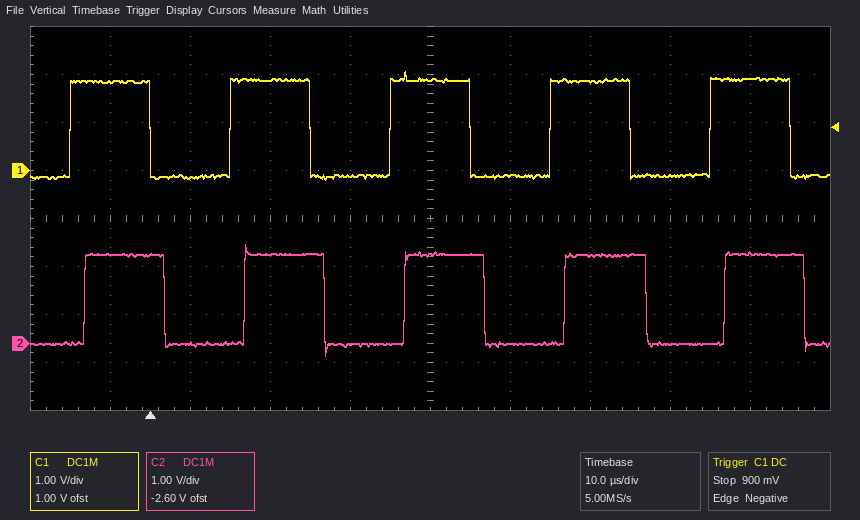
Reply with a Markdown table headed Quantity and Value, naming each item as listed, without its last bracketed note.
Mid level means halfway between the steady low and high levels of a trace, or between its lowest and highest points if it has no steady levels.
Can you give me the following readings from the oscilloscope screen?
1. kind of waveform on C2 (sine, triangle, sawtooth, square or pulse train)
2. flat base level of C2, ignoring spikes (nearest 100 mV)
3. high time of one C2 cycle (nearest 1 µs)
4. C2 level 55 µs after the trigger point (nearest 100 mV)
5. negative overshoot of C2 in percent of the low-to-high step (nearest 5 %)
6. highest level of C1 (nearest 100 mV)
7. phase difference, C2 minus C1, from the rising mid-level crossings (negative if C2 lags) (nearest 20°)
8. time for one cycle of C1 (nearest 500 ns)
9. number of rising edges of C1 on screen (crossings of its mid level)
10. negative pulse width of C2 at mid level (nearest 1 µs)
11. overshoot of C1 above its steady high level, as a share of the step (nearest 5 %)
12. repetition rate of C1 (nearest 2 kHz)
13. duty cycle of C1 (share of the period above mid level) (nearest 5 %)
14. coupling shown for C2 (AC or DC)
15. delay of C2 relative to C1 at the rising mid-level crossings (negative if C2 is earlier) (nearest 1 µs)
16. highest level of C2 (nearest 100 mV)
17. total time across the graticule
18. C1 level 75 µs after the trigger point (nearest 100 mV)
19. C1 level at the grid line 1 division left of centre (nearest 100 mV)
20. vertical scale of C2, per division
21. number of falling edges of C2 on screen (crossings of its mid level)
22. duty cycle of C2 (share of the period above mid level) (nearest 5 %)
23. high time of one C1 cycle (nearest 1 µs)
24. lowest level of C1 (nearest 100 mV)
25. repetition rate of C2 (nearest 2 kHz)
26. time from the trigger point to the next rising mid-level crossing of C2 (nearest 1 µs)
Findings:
| Quantity | Value |
|---|---|
| kind of waveform on C2 | square |
| flat base level of C2, ignoring spikes | 0.0 V |
| high time of one C2 cycle | 10 µs |
| C2 level 55 µs after the trigger point | 1.8 V |
| negative overshoot of C2 in percent of the low-to-high step | 15 % |
| highest level of C1 | 2.1 V |
| phase difference, C2 minus C1, from the rising mid-level crossings (negative if C2 lags) | -40° |
| time for one cycle of C1 | 20.0 µs |
| number of rising edges of C1 on screen | 5 |
| negative pulse width of C2 at mid level | 10 µs |
| overshoot of C1 above its steady high level, as a share of the step | 10 % |
| repetition rate of C1 | 50 kHz |
| duty cycle of C1 (share of the period above mid level) | 50 % |
| coupling shown for C2 | DC |
| delay of C2 relative to C1 at the rising mid-level crossings (negative if C2 is earlier) | +2 µs |
| highest level of C2 | 2.1 V |
| total time across the graticule | 100 µs |
| C1 level 75 µs after the trigger point | 1.9 V |
| C1 level at the grid line 1 division left of centre | -100 mV |
| vertical scale of C2, per division | 1 V |
| number of falling edges of C2 on screen | 5 |
| duty cycle of C2 (share of the period above mid level) | 50 % |
| high time of one C1 cycle | 10 µs |
| lowest level of C1 | -200 mV |
| repetition rate of C2 | 50 kHz |
| time from the trigger point to the next rising mid-level crossing of C2 | 12 µs |
